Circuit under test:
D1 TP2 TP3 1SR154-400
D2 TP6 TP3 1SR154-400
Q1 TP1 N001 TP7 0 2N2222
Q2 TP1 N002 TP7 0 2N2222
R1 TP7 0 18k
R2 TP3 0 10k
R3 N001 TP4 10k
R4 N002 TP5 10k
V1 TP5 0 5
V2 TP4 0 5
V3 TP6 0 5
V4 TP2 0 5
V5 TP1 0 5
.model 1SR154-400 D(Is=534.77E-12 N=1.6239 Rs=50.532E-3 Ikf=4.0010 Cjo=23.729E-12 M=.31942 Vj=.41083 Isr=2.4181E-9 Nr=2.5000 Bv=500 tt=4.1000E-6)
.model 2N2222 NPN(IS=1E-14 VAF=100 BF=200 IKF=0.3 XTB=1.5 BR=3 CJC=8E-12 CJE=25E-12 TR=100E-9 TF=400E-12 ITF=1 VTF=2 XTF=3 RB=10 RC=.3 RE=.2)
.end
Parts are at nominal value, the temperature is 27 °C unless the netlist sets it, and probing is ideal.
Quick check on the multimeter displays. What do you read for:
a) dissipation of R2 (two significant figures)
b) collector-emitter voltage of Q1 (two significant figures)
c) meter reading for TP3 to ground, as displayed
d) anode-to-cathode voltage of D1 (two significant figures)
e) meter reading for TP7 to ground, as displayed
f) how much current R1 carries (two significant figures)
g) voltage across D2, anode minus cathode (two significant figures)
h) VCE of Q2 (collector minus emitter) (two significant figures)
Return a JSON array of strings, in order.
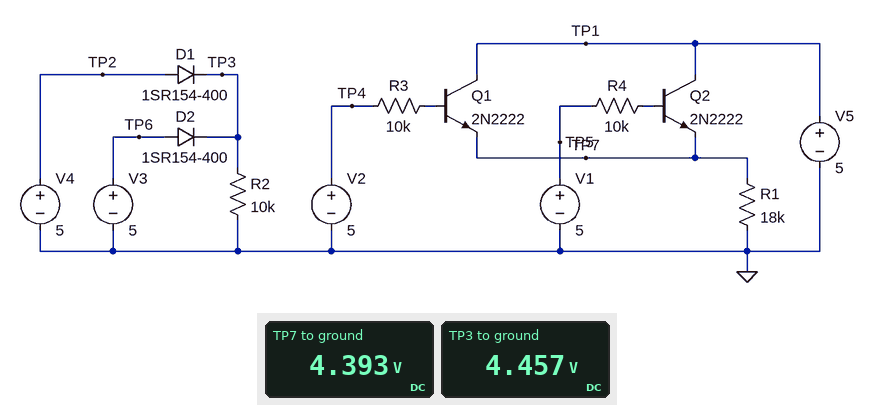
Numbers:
["2.0 mW", "610 mV", "4.457 V", "540 mV", "4.393 V", "240 µA", "540 mV", "610 mV"]
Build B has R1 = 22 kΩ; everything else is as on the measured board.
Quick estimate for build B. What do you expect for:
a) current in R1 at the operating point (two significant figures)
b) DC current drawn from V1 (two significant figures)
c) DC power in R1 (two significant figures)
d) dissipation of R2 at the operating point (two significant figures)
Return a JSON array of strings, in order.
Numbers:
["200 µA", "500 nA", "880 µW", "2.0 mW"]
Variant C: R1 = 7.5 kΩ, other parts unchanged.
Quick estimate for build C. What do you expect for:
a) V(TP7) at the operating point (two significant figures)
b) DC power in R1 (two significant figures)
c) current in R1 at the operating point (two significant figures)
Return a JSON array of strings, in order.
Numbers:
["4.4 V", "2.5 mW", "580 µA"]
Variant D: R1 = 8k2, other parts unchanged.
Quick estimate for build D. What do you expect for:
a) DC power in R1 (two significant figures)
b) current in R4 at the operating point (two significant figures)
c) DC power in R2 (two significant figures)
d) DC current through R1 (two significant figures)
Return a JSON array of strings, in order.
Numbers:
["2.3 mW", "1.3 µA", "2.0 mW", "530 µA"]
